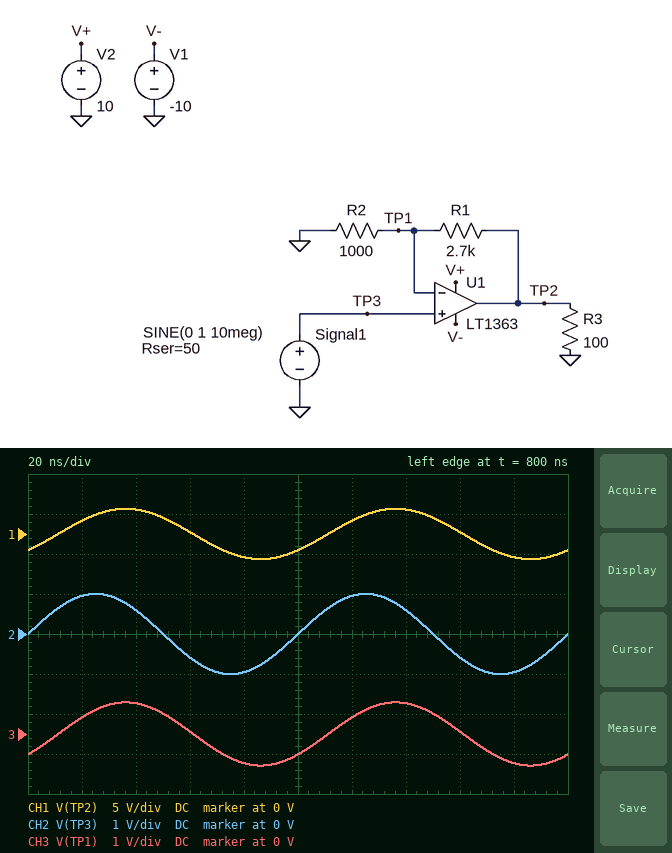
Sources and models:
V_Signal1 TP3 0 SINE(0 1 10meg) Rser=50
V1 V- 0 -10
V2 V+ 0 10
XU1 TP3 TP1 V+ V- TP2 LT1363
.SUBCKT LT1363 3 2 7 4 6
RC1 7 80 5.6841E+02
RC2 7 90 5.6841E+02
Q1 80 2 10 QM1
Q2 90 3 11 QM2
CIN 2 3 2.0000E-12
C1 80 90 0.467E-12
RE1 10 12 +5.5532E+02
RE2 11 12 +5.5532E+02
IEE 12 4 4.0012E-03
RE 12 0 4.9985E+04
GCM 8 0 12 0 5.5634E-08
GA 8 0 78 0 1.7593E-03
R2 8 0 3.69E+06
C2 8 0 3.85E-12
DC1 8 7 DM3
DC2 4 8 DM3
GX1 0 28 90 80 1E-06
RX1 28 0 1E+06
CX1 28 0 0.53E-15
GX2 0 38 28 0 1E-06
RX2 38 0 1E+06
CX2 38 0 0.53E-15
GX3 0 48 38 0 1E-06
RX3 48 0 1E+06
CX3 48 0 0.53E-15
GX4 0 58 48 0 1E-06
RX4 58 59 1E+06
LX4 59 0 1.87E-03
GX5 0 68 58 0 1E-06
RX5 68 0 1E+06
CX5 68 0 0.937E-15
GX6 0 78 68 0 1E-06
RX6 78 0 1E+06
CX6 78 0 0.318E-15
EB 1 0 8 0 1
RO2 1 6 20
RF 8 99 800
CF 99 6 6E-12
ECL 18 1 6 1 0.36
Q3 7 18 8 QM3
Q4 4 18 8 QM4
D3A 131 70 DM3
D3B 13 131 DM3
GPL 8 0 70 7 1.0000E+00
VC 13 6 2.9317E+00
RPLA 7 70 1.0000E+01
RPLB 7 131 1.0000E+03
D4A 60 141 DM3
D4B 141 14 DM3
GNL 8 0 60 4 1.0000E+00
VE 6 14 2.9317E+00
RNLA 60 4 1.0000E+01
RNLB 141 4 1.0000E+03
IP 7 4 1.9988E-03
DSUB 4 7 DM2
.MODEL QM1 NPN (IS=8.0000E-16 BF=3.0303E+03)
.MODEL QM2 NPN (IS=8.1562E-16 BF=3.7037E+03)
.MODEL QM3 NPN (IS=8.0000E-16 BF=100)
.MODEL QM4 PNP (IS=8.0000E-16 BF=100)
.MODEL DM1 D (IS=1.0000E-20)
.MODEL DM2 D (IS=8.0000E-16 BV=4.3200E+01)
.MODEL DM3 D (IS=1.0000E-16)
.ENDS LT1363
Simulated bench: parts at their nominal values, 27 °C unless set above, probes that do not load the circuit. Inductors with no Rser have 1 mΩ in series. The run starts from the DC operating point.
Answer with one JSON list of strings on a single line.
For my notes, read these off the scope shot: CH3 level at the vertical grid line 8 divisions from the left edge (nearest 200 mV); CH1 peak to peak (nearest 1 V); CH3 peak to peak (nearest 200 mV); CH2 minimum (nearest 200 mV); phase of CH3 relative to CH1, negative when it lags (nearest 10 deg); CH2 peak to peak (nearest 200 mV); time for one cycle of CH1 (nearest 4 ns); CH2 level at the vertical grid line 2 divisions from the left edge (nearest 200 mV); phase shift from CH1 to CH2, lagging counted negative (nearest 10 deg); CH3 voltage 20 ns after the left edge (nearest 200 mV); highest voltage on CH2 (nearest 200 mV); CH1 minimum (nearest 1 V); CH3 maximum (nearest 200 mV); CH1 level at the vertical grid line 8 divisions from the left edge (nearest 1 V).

["0 V", "6 V", "1.6 V", "-1.0 V", "0 deg", "2.0 V", "100 ns", "600 mV", "40 deg", "400 mV", "1.0 V", "-3 V", "800 mV", "0 V"]
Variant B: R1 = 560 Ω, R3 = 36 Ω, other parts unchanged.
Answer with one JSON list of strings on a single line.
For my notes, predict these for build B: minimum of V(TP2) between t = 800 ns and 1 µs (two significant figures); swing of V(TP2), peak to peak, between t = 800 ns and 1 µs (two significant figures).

["-1.4 V", "2.8 V"]
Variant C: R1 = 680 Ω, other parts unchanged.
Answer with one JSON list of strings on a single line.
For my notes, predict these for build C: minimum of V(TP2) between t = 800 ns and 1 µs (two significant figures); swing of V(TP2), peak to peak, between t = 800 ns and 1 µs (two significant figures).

["-1.6 V", "3.3 V"]
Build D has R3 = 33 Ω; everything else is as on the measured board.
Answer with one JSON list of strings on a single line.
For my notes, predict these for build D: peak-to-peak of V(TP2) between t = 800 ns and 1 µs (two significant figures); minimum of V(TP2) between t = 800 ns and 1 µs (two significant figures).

["4.8 V", "-2.4 V"]
